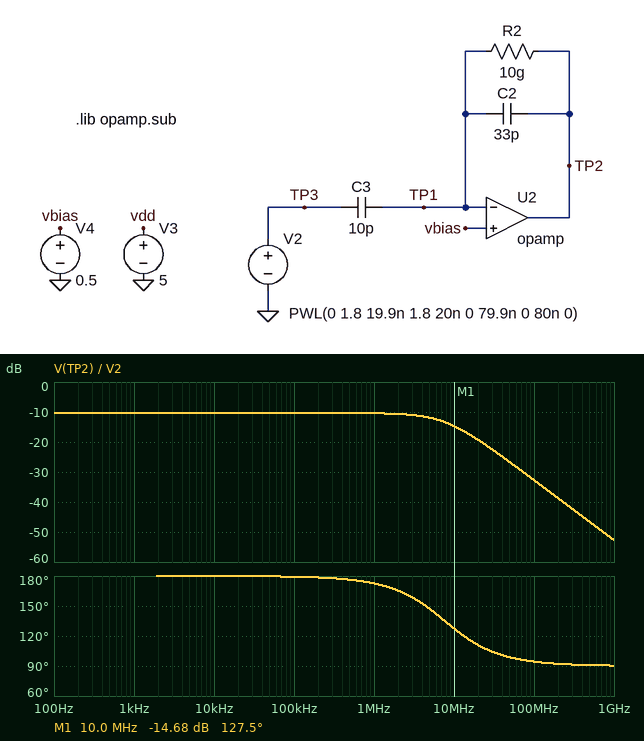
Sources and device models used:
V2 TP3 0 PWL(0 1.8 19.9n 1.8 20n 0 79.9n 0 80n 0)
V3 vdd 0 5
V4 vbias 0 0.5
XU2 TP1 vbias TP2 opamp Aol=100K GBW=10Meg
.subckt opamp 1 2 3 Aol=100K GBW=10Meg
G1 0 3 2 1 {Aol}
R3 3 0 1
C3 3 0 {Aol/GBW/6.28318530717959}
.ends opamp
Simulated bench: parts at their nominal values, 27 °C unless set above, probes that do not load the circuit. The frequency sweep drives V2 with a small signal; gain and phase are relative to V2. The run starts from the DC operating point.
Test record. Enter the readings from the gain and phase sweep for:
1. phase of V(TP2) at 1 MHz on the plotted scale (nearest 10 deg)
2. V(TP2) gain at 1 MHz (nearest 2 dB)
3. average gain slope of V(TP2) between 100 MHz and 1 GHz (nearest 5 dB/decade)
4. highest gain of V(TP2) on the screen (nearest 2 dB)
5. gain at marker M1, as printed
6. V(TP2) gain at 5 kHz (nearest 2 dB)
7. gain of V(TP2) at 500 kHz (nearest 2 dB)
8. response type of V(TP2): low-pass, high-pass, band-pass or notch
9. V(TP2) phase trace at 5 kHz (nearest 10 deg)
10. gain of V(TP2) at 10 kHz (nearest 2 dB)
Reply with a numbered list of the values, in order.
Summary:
1. 170 deg
2. -10 dB
3. -20 dB/decade
4. -10 dB
5. -14.68 dB
6. -10 dB
7. -10 dB
8. low-pass
9. 180 deg
10. -10 dB
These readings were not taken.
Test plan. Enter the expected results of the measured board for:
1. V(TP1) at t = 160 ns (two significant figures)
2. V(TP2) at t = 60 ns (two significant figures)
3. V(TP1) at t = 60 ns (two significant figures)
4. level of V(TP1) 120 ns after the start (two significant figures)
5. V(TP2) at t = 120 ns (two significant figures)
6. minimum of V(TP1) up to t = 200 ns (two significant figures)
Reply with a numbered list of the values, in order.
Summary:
1. 500 mV
2. 970 mV
3. 440 mV
4. 500 mV
5. 1.0 V
6. 82 mV
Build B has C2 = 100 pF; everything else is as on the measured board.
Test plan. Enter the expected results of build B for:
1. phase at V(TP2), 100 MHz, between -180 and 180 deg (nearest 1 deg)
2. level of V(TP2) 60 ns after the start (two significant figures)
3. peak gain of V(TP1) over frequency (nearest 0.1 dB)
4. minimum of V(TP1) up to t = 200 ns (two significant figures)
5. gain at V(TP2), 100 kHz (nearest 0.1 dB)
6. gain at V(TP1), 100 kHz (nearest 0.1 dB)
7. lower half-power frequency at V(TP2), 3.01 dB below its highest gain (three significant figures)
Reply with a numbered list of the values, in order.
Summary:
1. 95 deg
2. 660 mV
3. -20.8 dB
4. 340 mV
5. -20.0 dB
6. -60.0 dB
7. 159 mHz
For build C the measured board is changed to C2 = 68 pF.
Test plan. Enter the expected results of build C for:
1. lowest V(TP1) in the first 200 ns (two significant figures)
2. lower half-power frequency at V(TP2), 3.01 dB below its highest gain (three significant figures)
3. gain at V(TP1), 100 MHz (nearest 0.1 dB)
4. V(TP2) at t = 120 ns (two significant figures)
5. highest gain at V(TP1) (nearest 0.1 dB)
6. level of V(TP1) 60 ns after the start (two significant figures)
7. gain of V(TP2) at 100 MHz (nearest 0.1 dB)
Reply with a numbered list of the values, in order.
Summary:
1. 270 mV
2. 234 mHz
3. -17.9 dB
4. 760 mV
5. -17.8 dB
6. 470 mV
7. -37.9 dB
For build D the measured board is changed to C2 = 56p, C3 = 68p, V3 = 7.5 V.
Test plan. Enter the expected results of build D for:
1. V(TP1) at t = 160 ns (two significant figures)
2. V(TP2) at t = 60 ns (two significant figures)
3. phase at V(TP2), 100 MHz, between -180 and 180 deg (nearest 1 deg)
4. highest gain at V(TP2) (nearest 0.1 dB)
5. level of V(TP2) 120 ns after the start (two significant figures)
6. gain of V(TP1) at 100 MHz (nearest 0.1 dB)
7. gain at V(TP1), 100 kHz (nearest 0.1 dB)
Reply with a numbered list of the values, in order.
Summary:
1. 480 mV
2. 2.0 V
3. 93 deg
4. 1.7 dB
5. 2.6 V
6. -5.2 dB
7. -38.3 dB
